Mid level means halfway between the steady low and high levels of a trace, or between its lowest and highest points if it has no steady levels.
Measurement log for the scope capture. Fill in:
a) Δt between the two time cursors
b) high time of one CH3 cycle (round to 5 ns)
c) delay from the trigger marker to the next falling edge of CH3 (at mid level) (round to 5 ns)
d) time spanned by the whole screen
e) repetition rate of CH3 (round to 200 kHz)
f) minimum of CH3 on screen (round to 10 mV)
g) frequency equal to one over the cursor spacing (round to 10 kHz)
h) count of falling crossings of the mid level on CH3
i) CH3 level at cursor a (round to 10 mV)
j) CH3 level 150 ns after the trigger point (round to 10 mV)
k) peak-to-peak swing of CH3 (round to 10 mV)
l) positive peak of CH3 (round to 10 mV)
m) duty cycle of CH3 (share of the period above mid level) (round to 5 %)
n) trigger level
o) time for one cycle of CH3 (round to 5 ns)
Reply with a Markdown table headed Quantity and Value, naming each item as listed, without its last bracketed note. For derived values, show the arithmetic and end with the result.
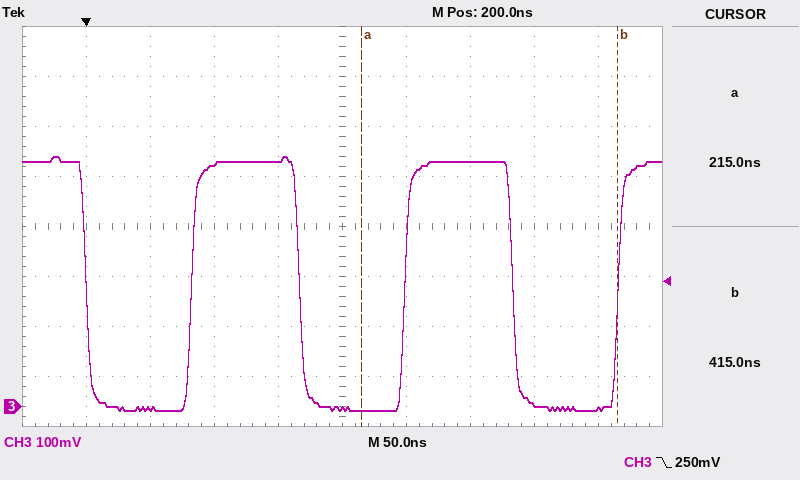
| Quantity | Value |
|---|---|
| Δt between the two time cursors | 415 ns − (215 ns) = 200 ns |
| high time of one CH3 cycle | 85 ns |
| delay from the trigger marker to the next falling edge of CH3 (at mid level) | 165 ns |
| time spanned by the whole screen | 500 ns |
| repetition rate of CH3 | 1 / 165 ns ≈ 6.06 MHz, so 6.0 MHz to the nearest 200 kHz |
| minimum of CH3 on screen | -10 mV |
| frequency equal to one over the cursor spacing | 1 / 200 ns ≈ 5.00 MHz |
| count of falling crossings of the mid level on CH3 | 3 |
| CH3 level at cursor a | -10 mV |
| CH3 level 150 ns after the trigger point | 490 mV |
| peak-to-peak swing of CH3 | 500 mV − (-10 mV) = 510 mV |
| positive peak of CH3 | 500 mV |
| duty cycle of CH3 (share of the period above mid level) | 85 ns / 165 ns ≈ 51.5 %, so 50 % to the nearest 5 % |
| trigger level | 250 mV |
| time for one cycle of CH3 | 165 ns |
